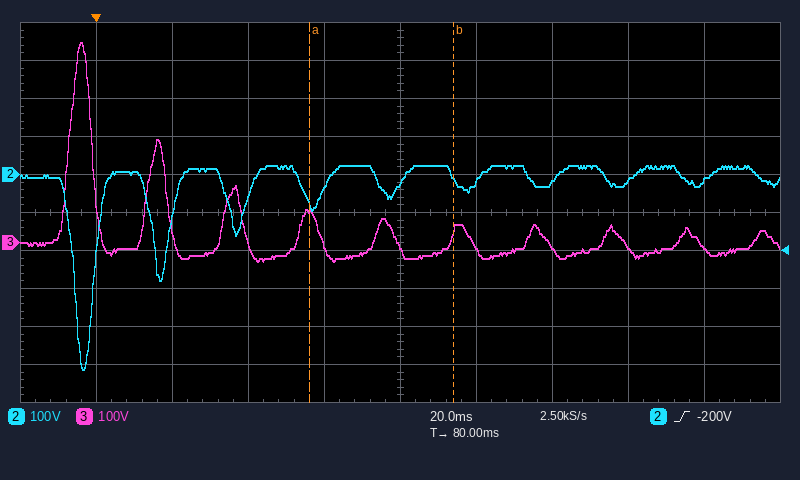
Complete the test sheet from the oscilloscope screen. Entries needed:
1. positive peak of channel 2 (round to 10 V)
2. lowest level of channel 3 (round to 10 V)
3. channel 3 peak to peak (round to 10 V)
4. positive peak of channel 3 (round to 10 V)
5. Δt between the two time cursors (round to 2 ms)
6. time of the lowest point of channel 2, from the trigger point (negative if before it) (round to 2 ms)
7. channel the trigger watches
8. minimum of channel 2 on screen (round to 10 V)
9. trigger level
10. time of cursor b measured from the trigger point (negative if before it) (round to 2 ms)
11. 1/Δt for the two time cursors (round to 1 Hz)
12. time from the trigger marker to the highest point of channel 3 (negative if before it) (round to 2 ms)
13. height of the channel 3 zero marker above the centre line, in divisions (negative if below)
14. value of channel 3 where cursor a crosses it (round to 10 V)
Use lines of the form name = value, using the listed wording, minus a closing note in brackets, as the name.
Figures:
positive peak of channel 2 = 20 V
lowest level of channel 3 = -50 V
channel 3 peak to peak = 580 V
positive peak of channel 3 = 530 V
Δt between the two time cursors = 38 ms
time of the lowest point of channel 2, from the trigger point (negative if before it) = -4 ms
channel the trigger watches = channel 2
minimum of channel 2 on screen = -510 V
trigger level = -200 V
time of cursor b measured from the trigger point (negative if before it) = +94 ms
1/Δt for the two time cursors = 26 Hz
time from the trigger marker to the highest point of channel 3 (negative if before it) = -4 ms
height of the channel 3 zero marker above the centre line, in divisions = -0.8 div
value of channel 3 where cursor a crosses it = 80 V
